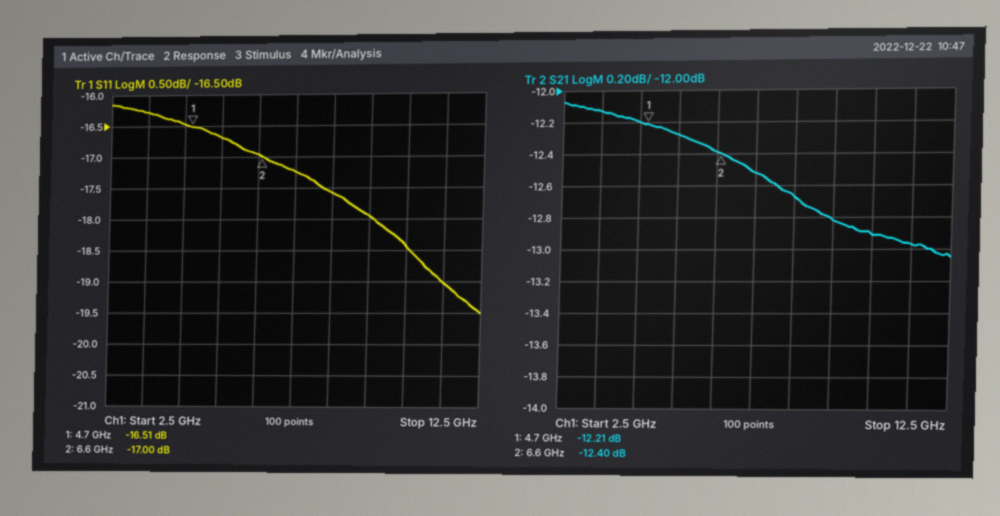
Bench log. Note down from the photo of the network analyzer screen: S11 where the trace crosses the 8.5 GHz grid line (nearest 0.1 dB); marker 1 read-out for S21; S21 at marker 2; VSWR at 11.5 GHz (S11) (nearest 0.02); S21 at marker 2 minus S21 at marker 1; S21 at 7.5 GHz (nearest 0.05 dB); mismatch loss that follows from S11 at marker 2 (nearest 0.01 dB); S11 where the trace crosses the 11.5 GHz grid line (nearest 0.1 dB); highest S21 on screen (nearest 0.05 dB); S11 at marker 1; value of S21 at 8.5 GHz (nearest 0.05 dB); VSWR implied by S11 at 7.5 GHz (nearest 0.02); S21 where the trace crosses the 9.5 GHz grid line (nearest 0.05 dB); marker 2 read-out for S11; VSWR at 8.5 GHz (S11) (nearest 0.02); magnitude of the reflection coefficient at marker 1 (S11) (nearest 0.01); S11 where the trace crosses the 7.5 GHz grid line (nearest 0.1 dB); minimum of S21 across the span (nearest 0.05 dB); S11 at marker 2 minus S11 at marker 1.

-17.6 dB
-12.21 dB
-12.40 dB
1.26
-0.19 dB
-12.50 dB
0.09 dB
-19.0 dB
-12.05 dB
-16.51 dB
-12.65 dB
1.32
-12.80 dB
-17.00 dB
1.30
0.15
-17.2 dB
-13.05 dB
-0.49 dB
